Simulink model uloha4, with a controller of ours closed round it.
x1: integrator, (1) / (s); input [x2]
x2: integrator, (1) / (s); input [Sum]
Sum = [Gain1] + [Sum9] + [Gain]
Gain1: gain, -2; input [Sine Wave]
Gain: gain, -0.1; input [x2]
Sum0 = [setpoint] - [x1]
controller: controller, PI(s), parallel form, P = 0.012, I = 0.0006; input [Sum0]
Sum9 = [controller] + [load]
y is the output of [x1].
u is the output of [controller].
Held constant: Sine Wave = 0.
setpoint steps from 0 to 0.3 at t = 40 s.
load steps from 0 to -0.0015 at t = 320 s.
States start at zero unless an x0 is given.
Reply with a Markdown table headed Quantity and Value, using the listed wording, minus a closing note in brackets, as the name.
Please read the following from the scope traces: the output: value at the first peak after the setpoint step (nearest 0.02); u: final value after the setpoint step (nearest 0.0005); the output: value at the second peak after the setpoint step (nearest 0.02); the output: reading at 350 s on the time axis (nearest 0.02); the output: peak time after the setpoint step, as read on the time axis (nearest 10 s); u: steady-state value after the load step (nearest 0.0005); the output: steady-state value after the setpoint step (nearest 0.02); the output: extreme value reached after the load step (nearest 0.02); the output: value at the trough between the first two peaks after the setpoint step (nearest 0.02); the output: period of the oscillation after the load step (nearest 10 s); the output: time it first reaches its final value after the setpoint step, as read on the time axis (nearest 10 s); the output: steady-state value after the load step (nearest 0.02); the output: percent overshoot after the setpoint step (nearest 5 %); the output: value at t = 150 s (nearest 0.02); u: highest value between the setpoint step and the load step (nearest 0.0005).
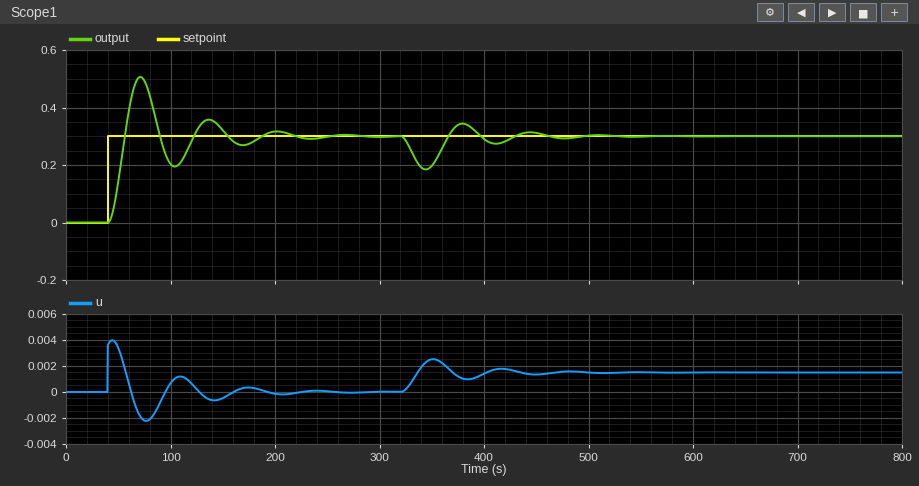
| Quantity | Value |
|---|---|
| the output: value at the first peak after the setpoint step | 0.50 |
| u: final value after the setpoint step | 0.0000 |
| the output: value at the second peak after the setpoint step | 0.36 |
| the output: reading at 350 s on the time axis | 0.20 |
| the output: peak time after the setpoint step, as read on the time axis | 70 s |
| u: steady-state value after the load step | 0.0015 |
| the output: steady-state value after the setpoint step | 0.30 |
| the output: extreme value reached after the load step | 0.18 |
| the output: value at the trough between the first two peaks after the setpoint step | 0.20 |
| the output: period of the oscillation after the load step | 70 s |
| the output: time it first reaches its final value after the setpoint step, as read on the time axis | 60 s |
| the output: steady-state value after the load step | 0.30 |
| the output: percent overshoot after the setpoint step | 70 % |
| the output: value at t = 150 s | 0.32 |
| u: highest value between the setpoint step and the load step | 0.0040 |
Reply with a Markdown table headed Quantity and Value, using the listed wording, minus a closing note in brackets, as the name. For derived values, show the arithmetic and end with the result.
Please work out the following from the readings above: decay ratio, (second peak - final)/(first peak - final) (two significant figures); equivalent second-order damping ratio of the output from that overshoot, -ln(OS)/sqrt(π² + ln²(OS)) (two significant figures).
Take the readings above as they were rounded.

| Quantity | Value |
|---|---|
| decay ratio, (second peak - final)/(first peak - final) | (0.36 - 0.3) / (0.5 - 0.3) = 0.30 |
| equivalent second-order damping ratio of the output from that overshoot, -ln(OS)/sqrt(π² + ln²(OS)) | ln(0.7) = -0.357; 0.357 / sqrt(9.870 + 0.127) = 0.11 |
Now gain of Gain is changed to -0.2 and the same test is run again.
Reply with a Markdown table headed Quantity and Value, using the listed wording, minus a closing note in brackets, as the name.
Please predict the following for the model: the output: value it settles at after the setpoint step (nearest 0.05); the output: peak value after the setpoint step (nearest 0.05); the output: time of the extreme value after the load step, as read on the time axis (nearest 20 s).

| Quantity | Value |
|---|---|
| the output: value it settles at after the setpoint step | 0.30 |
| the output: peak value after the setpoint step | 0.45 |
| the output: time of the extreme value after the load step, as read on the time axis | 340 s |
